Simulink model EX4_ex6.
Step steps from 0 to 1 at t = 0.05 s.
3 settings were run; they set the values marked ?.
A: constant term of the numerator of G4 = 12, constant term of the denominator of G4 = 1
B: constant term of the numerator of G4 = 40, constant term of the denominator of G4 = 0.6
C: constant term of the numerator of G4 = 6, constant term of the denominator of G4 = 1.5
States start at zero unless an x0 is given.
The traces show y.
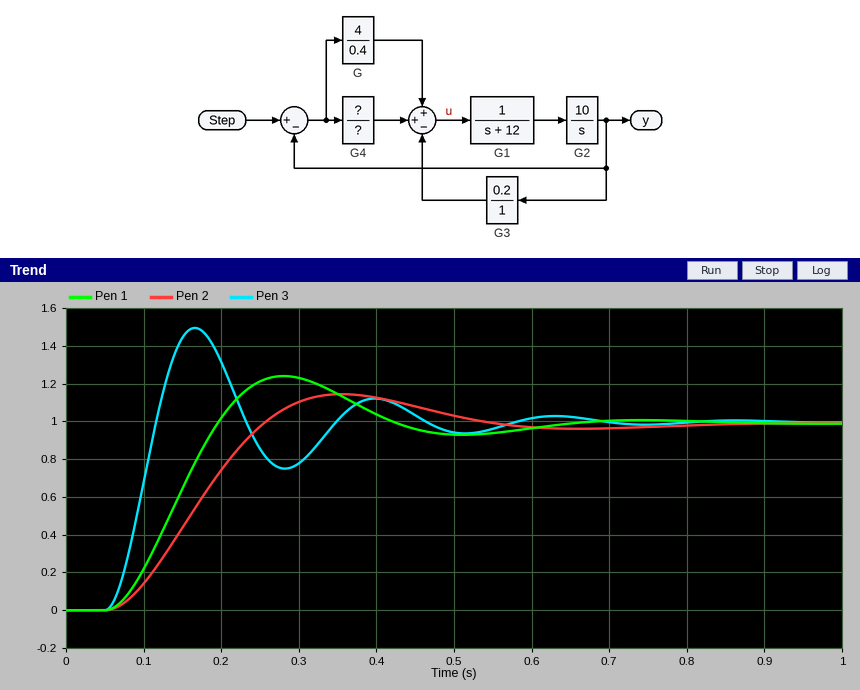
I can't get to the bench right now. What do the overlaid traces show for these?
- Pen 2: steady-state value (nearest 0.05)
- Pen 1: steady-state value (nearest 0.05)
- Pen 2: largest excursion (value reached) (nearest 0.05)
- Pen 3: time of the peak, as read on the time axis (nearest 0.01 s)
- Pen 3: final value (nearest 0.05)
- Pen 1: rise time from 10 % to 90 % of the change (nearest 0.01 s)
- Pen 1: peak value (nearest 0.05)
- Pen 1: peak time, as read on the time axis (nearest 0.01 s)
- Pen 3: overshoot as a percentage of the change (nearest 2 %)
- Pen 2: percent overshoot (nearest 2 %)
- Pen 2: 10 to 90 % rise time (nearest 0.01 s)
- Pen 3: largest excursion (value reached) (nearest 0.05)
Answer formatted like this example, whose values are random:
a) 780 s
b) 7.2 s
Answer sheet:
a) 1.00
b) 1.00
c) 1.15
d) 0.17 s
e) 1.00
f) 0.10 s
g) 1.25
h) 0.28 s
i) 50 %
j) 16 %
k) 0.14 s
l) 1.50
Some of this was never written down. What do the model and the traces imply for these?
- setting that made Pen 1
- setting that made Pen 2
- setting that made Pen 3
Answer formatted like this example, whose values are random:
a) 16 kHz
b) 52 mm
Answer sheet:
a) A
b) C
c) B
